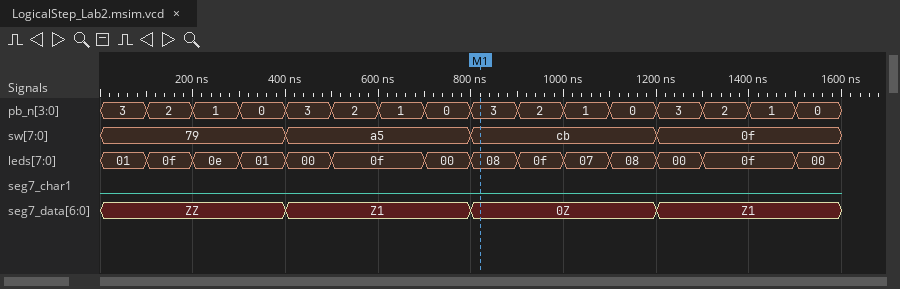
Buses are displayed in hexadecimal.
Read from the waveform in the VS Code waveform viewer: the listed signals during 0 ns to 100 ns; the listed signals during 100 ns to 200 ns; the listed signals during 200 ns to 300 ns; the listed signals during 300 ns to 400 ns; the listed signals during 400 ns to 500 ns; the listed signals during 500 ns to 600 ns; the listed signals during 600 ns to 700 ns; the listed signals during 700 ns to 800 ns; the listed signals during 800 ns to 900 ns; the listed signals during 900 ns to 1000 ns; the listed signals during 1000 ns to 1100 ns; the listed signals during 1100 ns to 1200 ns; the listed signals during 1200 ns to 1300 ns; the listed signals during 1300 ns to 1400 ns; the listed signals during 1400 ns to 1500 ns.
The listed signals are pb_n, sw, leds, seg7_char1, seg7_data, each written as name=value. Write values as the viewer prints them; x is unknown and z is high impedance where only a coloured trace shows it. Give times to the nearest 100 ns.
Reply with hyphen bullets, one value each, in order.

- pb_n=3, sw=79, leds=01, seg7_char1=0, seg7_data=ZZ
- pb_n=2, sw=79, leds=0f, seg7_char1=0, seg7_data=ZZ
- pb_n=1, sw=79, leds=0e, seg7_char1=0, seg7_data=ZZ
- pb_n=0, sw=79, leds=01, seg7_char1=0, seg7_data=ZZ
- pb_n=3, sw=a5, leds=00, seg7_char1=0, seg7_data=Z1
- pb_n=2, sw=a5, leds=0f, seg7_char1=0, seg7_data=Z1
- pb_n=1, sw=a5, leds=0f, seg7_char1=0, seg7_data=Z1
- pb_n=0, sw=a5, leds=00, seg7_char1=0, seg7_data=Z1
- pb_n=3, sw=cb, leds=08, seg7_char1=0, seg7_data=0Z
- pb_n=2, sw=cb, leds=0f, seg7_char1=0, seg7_data=0Z
- pb_n=1, sw=cb, leds=07, seg7_char1=0, seg7_data=0Z
- pb_n=0, sw=cb, leds=08, seg7_char1=0, seg7_data=0Z
- pb_n=3, sw=0f, leds=00, seg7_char1=0, seg7_data=Z1
- pb_n=2, sw=0f, leds=0f, seg7_char1=0, seg7_data=Z1
- pb_n=1, sw=0f, leds=0f, seg7_char1=0, seg7_data=Z1
